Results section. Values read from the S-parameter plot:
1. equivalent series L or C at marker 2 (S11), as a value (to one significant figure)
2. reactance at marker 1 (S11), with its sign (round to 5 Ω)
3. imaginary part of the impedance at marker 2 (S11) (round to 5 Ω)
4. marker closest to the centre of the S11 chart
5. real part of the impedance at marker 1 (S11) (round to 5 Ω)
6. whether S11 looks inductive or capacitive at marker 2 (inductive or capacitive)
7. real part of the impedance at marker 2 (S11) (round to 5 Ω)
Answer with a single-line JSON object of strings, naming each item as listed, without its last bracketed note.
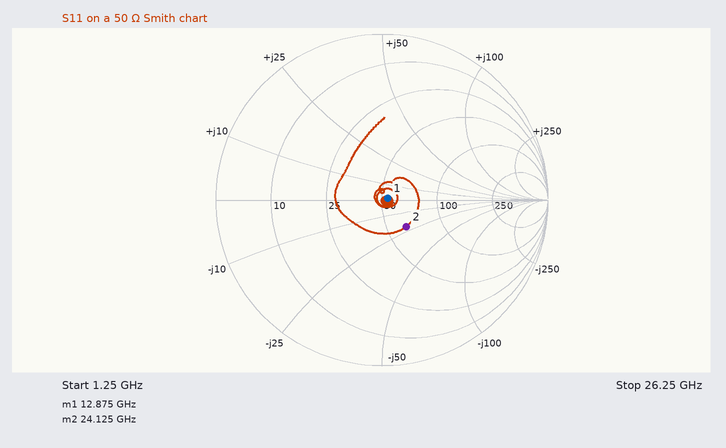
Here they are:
{"equivalent series L or C at marker 2 (S11), as a value": "300 fF", "reactance at marker 1 (S11), with its sign": "0 Ω", "imaginary part of the impedance at marker 2 (S11)": "-20 Ω", "marker closest to the centre of the S11 chart": "marker 1", "real part of the impedance at marker 1 (S11)": "55 Ω", "whether S11 looks inductive or capacitive at marker 2": "capacitive", "real part of the impedance at marker 2 (S11)": "65 Ω"}
